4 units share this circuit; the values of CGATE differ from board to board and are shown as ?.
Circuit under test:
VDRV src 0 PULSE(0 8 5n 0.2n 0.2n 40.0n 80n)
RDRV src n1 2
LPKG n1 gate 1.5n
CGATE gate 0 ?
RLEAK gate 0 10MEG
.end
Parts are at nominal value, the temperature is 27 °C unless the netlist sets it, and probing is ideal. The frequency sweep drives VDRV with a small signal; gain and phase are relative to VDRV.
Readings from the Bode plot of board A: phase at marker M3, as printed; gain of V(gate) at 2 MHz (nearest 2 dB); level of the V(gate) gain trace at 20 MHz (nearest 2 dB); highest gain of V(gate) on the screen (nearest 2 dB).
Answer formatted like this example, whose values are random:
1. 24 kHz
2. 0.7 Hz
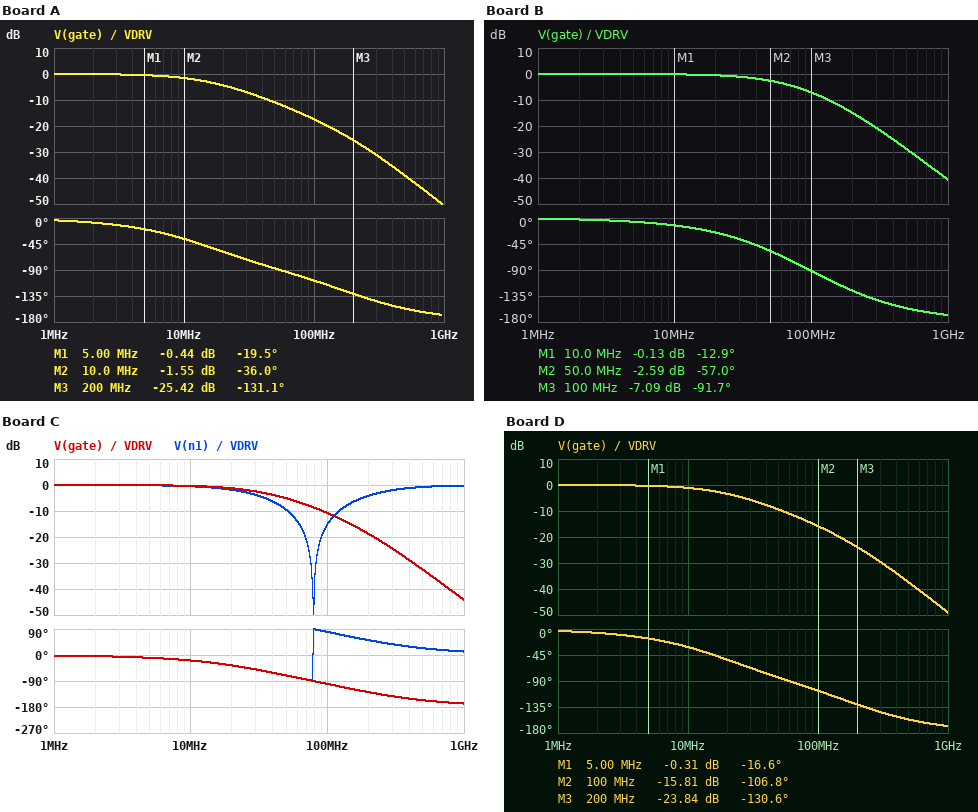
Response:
1. -131.1 deg
2. 0 dB
3. -4 dB
4. 0 dB
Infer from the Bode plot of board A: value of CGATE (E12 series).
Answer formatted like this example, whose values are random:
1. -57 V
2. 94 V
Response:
1. 5.6 nF
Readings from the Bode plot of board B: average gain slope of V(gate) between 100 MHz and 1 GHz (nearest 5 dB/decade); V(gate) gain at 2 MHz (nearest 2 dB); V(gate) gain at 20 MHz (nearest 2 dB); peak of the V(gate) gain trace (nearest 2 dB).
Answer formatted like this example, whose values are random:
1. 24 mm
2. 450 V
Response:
1. -35 dB/decade
2. 0 dB
3. 0 dB
4. 0 dB
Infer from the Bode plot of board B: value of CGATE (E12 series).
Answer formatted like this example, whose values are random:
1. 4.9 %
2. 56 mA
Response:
1. 1.8 nF
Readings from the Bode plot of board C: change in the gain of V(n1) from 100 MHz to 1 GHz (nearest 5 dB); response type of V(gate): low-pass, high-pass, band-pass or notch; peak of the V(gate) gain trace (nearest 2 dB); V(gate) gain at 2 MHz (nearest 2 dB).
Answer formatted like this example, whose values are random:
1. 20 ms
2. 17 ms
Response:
1. 15 dB
2. low-pass
3. 0 dB
4. 0 dB
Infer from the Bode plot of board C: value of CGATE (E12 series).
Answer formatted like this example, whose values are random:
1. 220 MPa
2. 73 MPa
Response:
1. 2.7 nF
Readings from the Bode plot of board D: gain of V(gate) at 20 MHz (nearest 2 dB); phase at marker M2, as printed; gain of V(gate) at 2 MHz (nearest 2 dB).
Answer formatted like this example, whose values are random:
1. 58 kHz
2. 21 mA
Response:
1. -4 dB
2. -106.8 deg
3. 0 dB
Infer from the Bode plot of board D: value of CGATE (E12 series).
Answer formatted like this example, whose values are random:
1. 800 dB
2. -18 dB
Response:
1. 4.7 nF
